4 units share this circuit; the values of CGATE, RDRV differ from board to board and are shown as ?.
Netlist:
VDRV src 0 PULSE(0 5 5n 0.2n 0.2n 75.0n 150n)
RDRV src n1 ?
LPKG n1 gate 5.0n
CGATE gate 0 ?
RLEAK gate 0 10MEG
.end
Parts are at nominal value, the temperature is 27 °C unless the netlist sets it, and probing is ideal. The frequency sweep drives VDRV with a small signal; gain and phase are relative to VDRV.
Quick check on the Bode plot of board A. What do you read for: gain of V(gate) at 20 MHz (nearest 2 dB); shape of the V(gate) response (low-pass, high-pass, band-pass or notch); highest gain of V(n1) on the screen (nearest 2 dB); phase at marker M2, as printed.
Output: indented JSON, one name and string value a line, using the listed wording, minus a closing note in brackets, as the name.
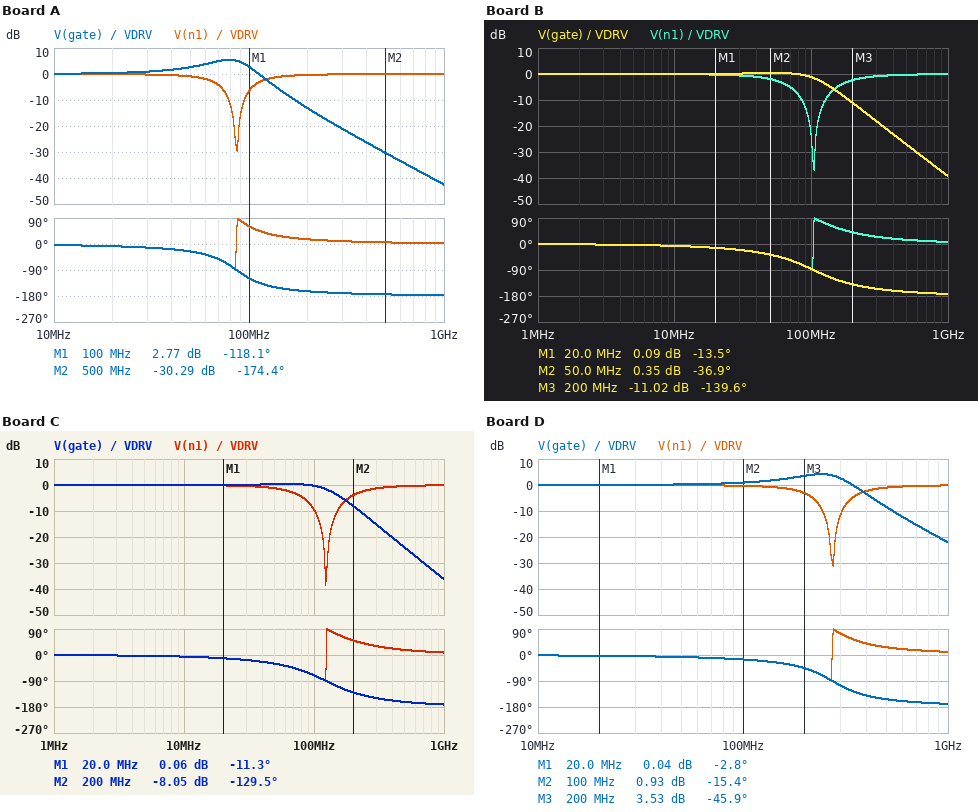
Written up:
{
  "gain of V(gate) at 20 MHz": "0 dB",
  "shape of the V(gate) response": "low-pass",
  "highest gain of V(n1) on the screen": "0 dB",
  "phase at marker M2, as printed": "-174.4 deg"
}
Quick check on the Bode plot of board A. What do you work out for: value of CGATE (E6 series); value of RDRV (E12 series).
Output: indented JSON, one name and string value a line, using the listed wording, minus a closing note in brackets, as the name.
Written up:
{
  "value of CGATE": "680 pF",
  "value of RDRV": "1.5 Ω"
}
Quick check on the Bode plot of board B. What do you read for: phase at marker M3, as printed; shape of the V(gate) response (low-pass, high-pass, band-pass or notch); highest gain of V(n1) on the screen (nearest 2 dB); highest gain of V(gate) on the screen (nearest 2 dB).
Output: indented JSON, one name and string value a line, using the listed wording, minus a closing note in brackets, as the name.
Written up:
{
  "phase at marker M3, as printed": "-139.6 deg",
  "shape of the V(gate) response": "low-pass",
  "highest gain of V(n1) on the screen": "0 dB",
  "highest gain of V(gate) on the screen": "0 dB"
}
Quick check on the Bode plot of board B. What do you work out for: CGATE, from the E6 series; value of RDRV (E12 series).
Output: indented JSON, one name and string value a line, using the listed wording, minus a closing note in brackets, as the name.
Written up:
{
  "CGATE, from the E6 series": "470 pF",
  "value of RDRV": "3.9 Ω"
}
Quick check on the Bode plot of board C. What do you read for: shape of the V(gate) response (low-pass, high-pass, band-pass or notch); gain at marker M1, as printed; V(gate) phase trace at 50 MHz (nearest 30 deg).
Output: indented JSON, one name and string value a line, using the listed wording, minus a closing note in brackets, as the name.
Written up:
{
  "shape of the V(gate) response": "low-pass",
  "gain at marker M1, as printed": "0.06 dB",
  "V(gate) phase trace at 50 MHz": "-30 deg"
}
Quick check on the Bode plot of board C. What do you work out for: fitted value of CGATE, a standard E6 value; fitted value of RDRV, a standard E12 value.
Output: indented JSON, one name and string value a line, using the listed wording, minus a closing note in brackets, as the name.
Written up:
{
  "fitted value of CGATE, a standard E6 value": "330 pF",
  "fitted value of RDRV, a standard E12 value": "4.7 Ω"
}
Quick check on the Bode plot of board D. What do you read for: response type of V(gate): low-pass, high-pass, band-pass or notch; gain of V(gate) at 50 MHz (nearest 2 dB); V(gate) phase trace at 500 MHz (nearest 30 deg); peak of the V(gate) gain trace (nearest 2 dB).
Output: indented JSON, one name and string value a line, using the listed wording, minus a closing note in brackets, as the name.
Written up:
{
  "response type of V(gate): low-pass, high-pass, band-pass or notch": "low-pass",
  "gain of V(gate) at 50 MHz": "0 dB",
  "V(gate) phase trace at 500 MHz": "-150 deg",
  "peak of the V(gate) gain trace": "4 dB"
}
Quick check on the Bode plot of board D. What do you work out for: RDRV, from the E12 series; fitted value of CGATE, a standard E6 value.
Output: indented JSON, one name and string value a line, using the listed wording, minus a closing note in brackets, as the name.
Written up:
{
  "RDRV, from the E12 series": "5.6 Ω",
  "fitted value of CGATE, a standard E6 value": "68 pF"
}
